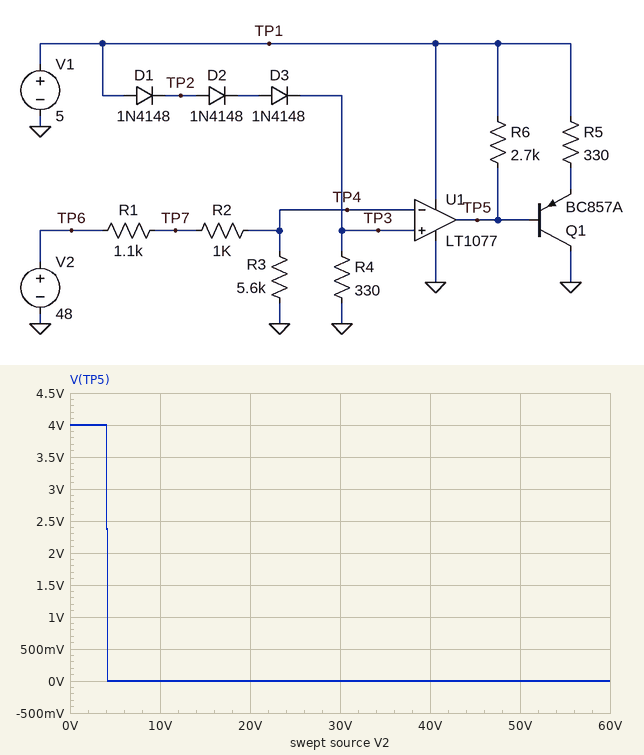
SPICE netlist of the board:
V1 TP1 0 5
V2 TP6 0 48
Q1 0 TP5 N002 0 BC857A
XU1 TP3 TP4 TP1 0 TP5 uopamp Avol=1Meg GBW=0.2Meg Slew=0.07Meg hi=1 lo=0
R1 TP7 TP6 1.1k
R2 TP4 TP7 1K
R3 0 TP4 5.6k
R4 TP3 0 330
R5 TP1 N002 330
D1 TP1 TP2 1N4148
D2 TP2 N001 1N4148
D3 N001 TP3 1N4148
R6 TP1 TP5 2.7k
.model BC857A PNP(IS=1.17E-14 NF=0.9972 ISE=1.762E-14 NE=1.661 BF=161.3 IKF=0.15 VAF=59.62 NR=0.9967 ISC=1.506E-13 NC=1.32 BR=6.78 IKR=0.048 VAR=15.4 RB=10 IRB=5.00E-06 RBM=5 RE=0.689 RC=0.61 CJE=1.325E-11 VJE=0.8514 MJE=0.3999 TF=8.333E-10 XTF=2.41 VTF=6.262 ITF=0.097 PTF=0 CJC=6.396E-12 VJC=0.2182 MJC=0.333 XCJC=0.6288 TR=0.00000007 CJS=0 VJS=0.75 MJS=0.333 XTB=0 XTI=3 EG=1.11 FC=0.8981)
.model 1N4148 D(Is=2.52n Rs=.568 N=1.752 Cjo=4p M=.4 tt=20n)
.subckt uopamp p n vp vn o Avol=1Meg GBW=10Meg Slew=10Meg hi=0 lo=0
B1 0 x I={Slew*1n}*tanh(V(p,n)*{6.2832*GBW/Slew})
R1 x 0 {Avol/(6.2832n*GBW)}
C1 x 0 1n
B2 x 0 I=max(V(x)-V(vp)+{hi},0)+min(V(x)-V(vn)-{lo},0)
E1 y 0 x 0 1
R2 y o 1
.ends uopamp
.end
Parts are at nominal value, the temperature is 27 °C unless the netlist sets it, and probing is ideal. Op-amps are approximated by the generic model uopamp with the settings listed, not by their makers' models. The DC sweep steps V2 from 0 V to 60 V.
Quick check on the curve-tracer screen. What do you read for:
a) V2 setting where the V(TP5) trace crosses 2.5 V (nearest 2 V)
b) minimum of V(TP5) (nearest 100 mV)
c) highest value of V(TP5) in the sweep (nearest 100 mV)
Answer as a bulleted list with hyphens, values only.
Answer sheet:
- 4 V
- 0 V
- 4.0 V
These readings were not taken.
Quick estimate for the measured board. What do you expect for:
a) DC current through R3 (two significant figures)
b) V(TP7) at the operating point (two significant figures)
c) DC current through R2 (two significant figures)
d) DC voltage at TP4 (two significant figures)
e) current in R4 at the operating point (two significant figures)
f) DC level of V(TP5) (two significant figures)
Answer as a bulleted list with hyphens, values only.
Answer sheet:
- 6.2 mA
- 41 V
- 6.2 mA
- 35 V
- 8.9 mA
- 1.9 mV
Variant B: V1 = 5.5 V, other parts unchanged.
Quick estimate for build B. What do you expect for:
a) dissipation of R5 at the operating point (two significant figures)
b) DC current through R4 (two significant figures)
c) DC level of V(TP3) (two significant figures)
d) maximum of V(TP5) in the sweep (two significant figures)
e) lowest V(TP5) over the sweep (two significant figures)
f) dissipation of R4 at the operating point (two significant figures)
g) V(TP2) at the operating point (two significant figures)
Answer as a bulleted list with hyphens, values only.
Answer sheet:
- 69 mW
- 10 mA
- 3.4 V
- 4.5 V
- 2.1 mV
- 35 mW
- 4.8 V
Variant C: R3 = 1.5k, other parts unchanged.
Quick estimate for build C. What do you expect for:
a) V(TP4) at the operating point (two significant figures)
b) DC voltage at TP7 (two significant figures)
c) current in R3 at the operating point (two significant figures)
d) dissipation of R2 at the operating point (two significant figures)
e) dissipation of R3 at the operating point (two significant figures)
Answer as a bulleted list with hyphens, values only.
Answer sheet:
- 20 V
- 33 V
- 13 mA
- 180 mW
- 270 mW
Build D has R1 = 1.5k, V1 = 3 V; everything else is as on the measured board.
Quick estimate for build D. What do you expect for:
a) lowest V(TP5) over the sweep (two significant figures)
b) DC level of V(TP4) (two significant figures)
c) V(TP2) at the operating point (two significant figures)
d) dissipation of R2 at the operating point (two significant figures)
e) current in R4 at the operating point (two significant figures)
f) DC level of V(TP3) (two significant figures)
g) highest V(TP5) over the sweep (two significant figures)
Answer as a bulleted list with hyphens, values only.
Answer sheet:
- 1.1 mV
- 33 V
- 2.4 V
- 35 mW
- 3.3 mA
- 1.1 V
- 2.0 V
